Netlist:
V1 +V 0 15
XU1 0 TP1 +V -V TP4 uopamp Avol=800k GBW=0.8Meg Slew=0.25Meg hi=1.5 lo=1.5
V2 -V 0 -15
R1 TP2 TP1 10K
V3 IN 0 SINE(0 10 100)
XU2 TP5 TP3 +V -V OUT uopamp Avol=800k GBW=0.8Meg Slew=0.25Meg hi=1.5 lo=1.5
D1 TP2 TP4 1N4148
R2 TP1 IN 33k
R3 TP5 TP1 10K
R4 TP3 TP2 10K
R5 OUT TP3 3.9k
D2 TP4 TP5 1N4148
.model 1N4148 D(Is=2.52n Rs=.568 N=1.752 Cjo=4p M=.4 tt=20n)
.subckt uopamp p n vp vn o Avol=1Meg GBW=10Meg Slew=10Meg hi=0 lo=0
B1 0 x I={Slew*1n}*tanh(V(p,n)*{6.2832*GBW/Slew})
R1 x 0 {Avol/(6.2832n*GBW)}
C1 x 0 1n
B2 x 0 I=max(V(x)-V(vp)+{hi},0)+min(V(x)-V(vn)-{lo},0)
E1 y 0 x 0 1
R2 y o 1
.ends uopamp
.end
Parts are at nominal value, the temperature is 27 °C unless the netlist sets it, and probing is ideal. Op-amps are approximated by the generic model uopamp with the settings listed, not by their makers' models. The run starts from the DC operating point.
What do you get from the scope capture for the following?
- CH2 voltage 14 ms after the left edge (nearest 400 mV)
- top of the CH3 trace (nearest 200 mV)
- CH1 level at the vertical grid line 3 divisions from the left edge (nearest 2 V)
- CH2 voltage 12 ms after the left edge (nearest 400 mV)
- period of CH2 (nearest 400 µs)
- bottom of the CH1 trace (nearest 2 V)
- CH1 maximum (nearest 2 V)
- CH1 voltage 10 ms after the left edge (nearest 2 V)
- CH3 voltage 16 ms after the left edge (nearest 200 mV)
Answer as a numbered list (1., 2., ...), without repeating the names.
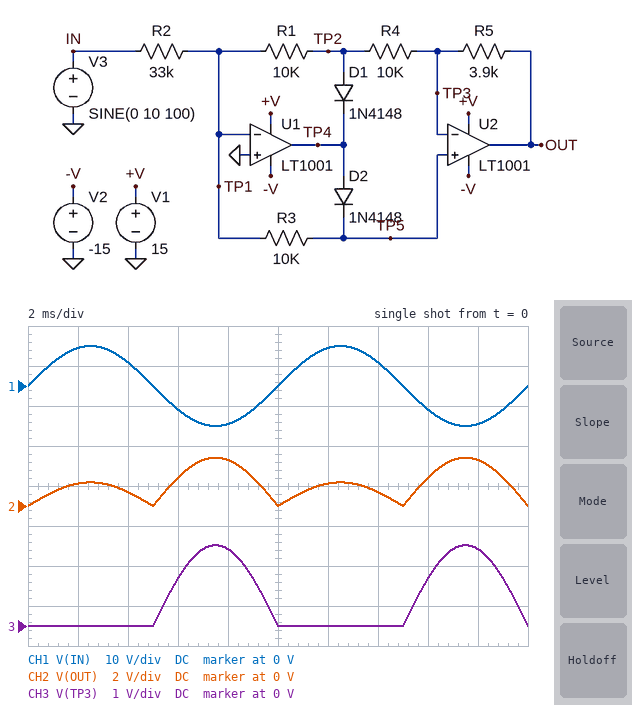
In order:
1. 800 mV
2. 2.0 V
3. -6 V
4. 1.2 V
5. 10.0 ms
6. -10 V
7. 10 V
8. 0 V
9. 1.2 V
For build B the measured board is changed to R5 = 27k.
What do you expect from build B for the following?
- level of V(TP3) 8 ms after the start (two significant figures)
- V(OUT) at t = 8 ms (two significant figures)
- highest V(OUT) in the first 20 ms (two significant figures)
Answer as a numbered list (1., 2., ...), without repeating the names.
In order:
1. 1.9 V
2. 4.5 V
3. 8.2 V
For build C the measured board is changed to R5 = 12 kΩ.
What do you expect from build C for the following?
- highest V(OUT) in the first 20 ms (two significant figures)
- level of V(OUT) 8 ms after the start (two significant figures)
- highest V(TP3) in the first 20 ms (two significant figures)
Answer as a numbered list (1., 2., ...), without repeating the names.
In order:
1. 3.6 V
2. 3.1 V
3. 2.0 V
